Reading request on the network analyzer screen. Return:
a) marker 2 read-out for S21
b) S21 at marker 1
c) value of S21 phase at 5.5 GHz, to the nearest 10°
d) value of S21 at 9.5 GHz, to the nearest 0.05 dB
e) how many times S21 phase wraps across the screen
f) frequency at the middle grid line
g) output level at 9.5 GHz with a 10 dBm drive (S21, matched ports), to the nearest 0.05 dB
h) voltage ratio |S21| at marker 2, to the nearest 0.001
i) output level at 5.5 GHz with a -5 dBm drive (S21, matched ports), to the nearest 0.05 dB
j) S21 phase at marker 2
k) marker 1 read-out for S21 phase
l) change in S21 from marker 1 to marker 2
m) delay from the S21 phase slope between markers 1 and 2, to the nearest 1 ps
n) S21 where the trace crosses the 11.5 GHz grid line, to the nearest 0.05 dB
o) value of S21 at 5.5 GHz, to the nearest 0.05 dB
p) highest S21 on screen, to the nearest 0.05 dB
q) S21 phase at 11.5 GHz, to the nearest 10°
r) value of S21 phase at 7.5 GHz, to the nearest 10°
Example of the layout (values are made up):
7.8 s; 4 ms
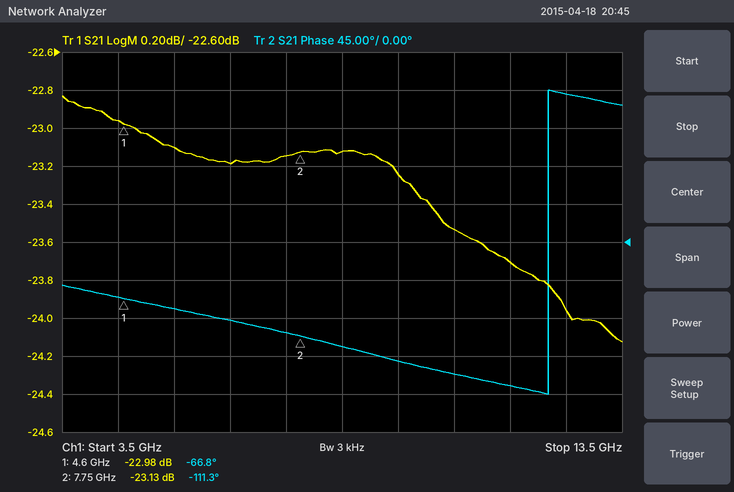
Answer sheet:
-23.13 dB; -22.98 dB; -80°; -23.25 dB; 1; 8.5 GHz; -13.25 dBm; 0.070; -28.10 dBm; -111.3°; -66.8°; -0.15 dB; 39 ps; -23.70 dB; -23.10 dB; -22.85 dB; -170°; -110°
